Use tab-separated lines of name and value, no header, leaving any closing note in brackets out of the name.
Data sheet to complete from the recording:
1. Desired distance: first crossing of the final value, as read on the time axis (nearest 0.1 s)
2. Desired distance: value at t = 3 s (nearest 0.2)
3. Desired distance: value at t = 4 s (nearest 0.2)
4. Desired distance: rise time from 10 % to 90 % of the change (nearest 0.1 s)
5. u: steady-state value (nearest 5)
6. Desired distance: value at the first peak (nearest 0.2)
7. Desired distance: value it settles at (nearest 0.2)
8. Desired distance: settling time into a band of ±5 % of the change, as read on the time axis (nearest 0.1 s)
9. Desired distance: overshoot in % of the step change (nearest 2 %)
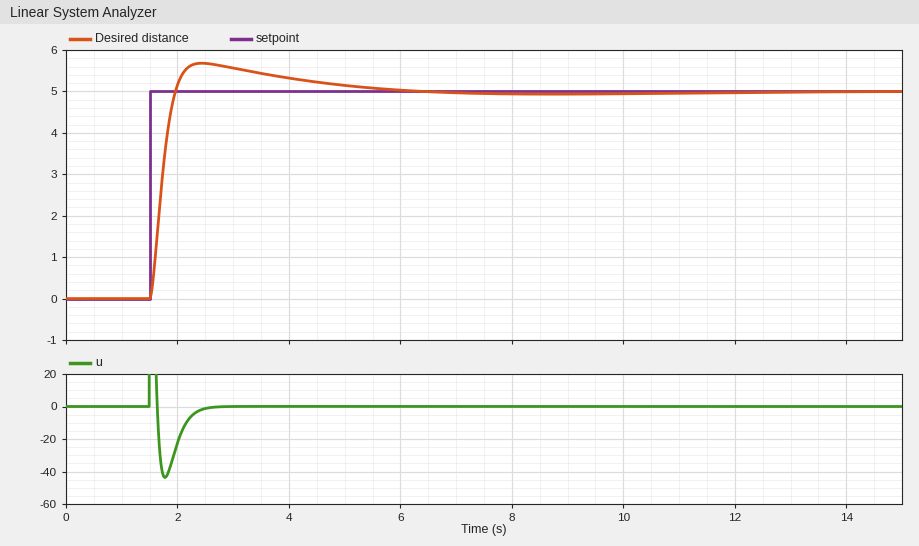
Desired distance: first crossing of the final value, as read on the time axis	2.0 s
Desired distance: value at t = 3 s	5.6
Desired distance: value at t = 4 s	5.4
Desired distance: rise time from 10 % to 90 % of the change	0.3 s
u: steady-state value	0
Desired distance: value at the first peak	5.6
Desired distance: value it settles at	5.0
Desired distance: settling time into a band of ±5 % of the change, as read on the time axis	4.4 s
Desired distance: overshoot in % of the step change	14 %
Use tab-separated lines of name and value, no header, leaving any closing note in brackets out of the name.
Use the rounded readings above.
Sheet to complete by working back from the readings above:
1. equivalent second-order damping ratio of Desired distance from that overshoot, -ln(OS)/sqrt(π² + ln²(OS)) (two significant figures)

equivalent second-order damping ratio of Desired distance from that overshoot, -ln(OS)/sqrt(π² + ln²(OS))	0.53
